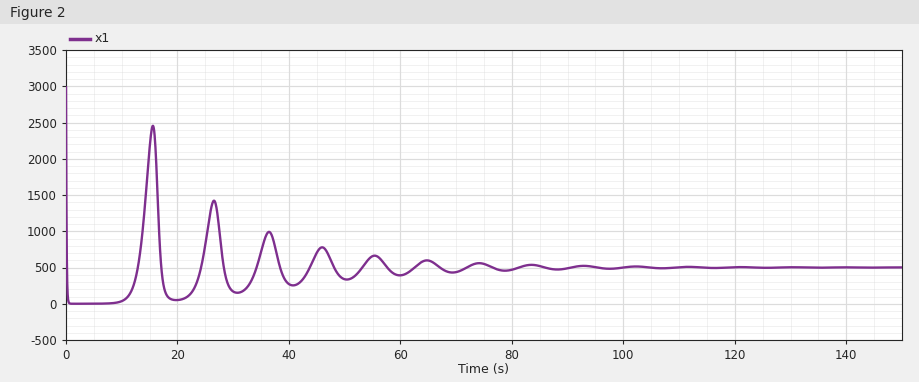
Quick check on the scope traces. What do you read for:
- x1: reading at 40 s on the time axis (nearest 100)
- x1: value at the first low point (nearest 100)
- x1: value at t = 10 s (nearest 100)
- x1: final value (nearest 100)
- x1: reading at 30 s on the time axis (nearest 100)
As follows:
300
0
0
500
200
